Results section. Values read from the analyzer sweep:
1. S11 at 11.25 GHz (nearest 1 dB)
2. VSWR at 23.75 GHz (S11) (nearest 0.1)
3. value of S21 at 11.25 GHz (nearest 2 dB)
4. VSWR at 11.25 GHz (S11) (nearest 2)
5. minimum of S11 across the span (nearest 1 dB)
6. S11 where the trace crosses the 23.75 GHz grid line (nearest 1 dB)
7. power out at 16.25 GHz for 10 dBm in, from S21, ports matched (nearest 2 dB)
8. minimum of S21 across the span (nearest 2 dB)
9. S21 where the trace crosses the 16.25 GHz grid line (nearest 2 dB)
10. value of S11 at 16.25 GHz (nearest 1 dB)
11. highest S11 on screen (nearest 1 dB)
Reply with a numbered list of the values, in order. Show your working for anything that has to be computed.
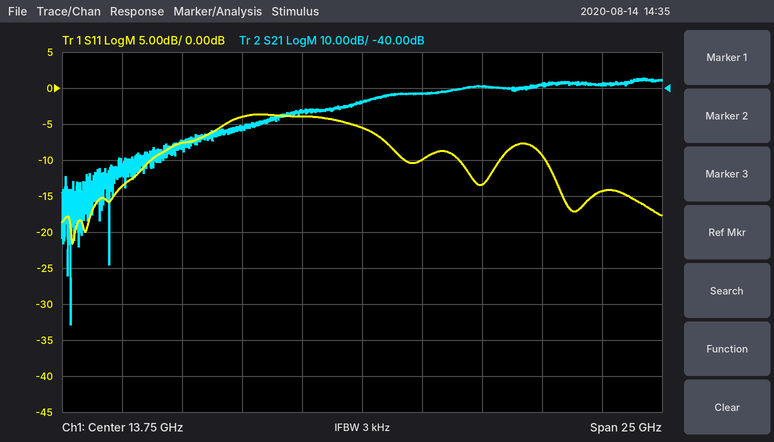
1. -4 dB
2. |Γ| = 10^(-14/20) = 0.1995; VSWR = (1 + 0.1995)/(1 − 0.1995) ≈ 1.5
3. -46 dB
4. |Γ| = 10^(-4/20) = 0.6310; VSWR = (1 + 0.6310)/(1 − 0.6310) ≈ 4
5. -22 dB
6. -14 dB
7. 10 dBm + (-42 dB) = -32 dBm
8. -106 dB
9. -42 dB
10. -10 dB
11. -4 dB
